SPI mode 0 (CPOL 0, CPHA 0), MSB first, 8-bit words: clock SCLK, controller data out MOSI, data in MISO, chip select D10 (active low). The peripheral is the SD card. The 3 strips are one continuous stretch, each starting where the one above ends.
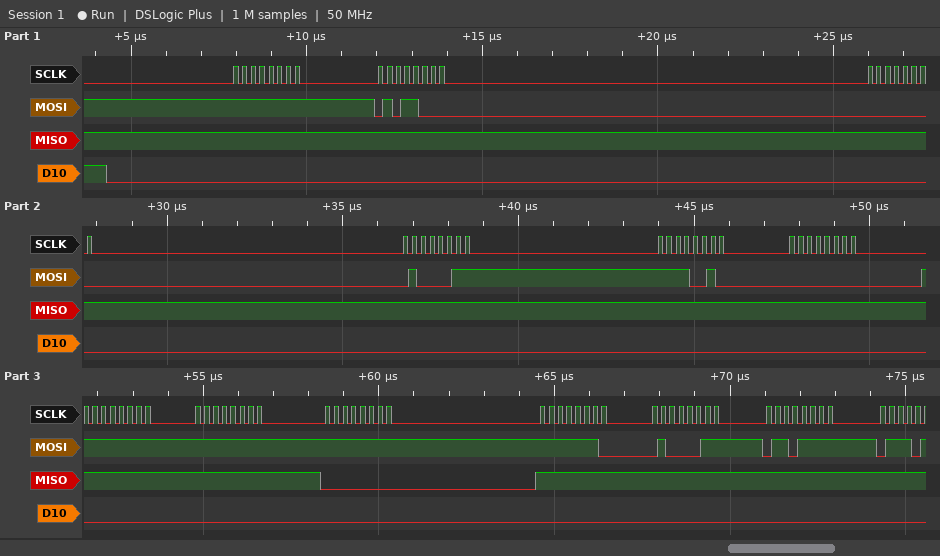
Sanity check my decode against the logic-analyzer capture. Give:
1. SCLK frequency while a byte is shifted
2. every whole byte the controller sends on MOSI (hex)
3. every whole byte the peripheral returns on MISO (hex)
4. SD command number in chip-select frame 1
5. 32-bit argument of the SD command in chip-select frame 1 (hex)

4 MHz
0xFF 0x58 0x00 0x43 0xF2 0x00 0xFF 0xFF 0xFF 0xFE 0x43 0x6F
0xFF 0xFF 0xFF 0xFF 0xFF 0xFF 0xFF 0xFF 0x00 0xFF 0xFF 0xFF
CMD24
0x0043F200
